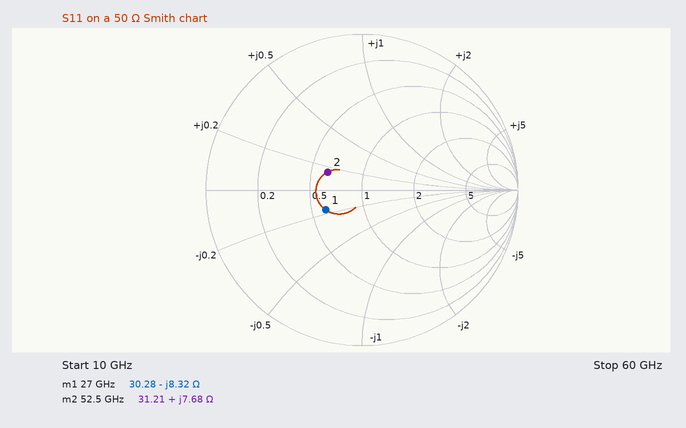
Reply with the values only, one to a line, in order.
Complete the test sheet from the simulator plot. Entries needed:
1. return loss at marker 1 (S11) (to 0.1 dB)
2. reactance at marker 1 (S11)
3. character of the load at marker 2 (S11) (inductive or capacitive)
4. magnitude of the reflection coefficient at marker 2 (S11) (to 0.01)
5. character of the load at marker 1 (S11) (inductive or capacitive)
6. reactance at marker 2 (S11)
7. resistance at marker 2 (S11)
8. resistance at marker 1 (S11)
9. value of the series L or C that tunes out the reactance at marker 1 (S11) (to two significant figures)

11.5 dB
-8.32 Ω
inductive
0.25
capacitive
+7.68 Ω
31.21 Ω
30.28 Ω
49 pH
